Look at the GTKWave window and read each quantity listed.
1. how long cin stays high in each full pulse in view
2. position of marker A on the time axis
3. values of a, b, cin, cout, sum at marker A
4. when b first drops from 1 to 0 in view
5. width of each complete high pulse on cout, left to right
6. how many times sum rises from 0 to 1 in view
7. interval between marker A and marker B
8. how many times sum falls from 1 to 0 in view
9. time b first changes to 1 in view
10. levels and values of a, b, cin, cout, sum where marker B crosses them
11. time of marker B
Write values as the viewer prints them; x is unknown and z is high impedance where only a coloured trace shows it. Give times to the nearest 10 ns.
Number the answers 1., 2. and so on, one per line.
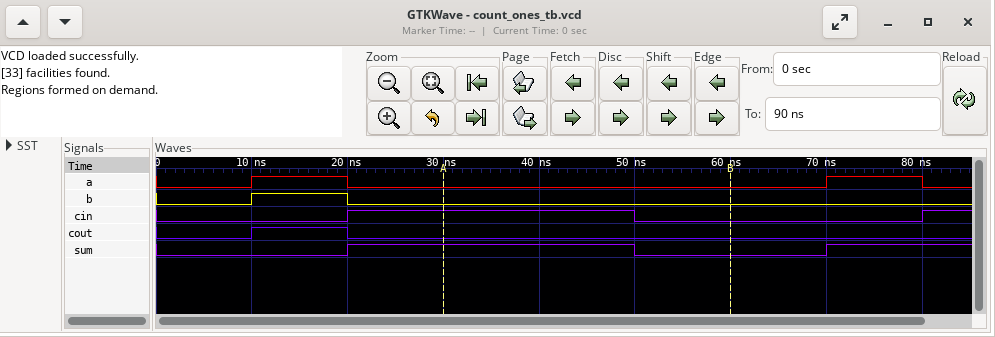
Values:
1. 30 ns
2. 30 ns
3. a=0, b=0, cin=1, cout=0, sum=1
4. 20 ns
5. 10 ns
6. 2
7. 30 ns
8. 1
9. 10 ns
10. a=0, b=0, cin=0, cout=0, sum=0
11. 60 ns
